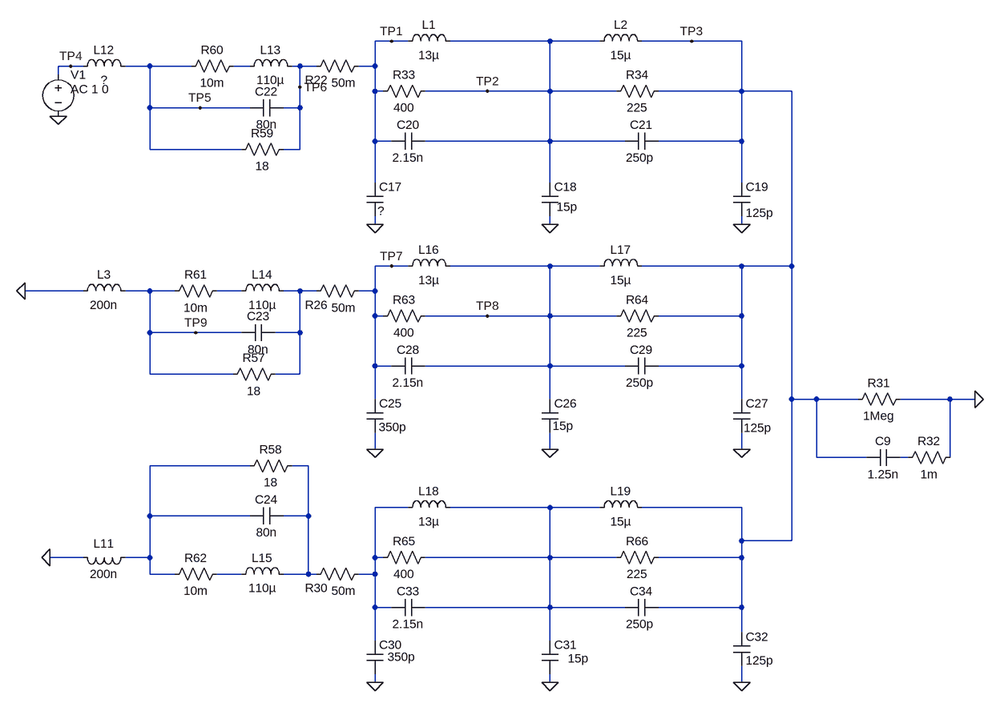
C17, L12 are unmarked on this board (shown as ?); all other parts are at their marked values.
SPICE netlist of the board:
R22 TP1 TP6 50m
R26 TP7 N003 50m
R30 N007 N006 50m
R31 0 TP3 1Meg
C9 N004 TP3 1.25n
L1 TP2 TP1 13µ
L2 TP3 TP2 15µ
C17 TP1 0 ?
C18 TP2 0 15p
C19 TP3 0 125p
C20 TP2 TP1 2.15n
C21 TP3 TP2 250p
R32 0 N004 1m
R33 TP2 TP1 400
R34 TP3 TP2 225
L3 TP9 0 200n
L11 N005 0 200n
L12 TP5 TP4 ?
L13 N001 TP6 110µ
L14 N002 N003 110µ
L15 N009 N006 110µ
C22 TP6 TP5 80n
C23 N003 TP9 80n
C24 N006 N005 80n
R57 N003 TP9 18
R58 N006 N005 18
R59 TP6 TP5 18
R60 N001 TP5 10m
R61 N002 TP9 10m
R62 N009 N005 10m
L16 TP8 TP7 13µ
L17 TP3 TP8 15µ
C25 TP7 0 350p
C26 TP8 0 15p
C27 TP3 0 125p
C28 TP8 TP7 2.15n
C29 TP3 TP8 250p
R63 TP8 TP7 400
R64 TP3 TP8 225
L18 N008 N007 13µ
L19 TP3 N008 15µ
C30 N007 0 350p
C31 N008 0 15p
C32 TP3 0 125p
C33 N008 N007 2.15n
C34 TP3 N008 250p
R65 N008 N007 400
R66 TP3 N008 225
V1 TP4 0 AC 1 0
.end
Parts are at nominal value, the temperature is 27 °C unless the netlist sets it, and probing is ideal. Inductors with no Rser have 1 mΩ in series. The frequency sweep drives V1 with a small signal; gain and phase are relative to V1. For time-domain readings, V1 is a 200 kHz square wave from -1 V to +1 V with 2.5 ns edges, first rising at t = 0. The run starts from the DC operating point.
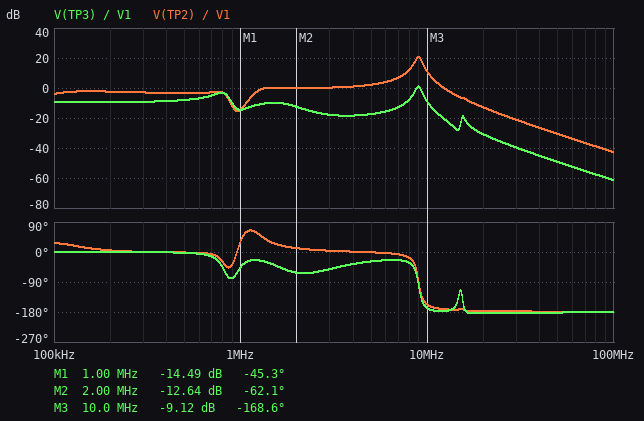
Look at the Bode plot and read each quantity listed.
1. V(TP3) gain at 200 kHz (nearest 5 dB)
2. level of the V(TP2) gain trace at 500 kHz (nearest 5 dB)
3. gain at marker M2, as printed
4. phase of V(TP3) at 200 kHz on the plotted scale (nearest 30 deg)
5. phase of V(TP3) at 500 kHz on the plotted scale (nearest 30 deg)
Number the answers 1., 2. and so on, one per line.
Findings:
1. -10 dB
2. -5 dB
3. -12.64 dB
4. 0 deg
5. 0 deg
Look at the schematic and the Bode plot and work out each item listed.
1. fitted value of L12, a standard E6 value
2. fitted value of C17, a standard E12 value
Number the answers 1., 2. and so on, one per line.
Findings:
1. 470 nH
2. 470 pF
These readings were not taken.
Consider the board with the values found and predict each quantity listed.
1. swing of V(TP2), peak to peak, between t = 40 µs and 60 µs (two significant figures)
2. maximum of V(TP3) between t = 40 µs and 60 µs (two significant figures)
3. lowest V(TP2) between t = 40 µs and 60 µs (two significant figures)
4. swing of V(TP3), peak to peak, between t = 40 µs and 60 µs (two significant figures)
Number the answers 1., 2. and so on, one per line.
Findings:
1. 5.2 V
2. 510 mV
3. -2.5 V
4. 1.0 V
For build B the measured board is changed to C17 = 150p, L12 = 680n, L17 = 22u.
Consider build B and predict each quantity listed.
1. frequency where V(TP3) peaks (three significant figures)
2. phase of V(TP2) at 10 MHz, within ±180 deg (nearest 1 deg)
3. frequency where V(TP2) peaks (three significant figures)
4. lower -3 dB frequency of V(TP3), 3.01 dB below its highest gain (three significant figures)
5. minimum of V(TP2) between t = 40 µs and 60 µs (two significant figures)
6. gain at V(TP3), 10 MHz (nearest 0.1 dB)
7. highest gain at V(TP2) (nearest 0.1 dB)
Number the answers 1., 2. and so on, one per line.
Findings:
1. 787 kHz
2. -68 deg
3. 10.2 MHz
4. 637 kHz
5. -2.4 V
6. -3.8 dB
7. 16.5 dB
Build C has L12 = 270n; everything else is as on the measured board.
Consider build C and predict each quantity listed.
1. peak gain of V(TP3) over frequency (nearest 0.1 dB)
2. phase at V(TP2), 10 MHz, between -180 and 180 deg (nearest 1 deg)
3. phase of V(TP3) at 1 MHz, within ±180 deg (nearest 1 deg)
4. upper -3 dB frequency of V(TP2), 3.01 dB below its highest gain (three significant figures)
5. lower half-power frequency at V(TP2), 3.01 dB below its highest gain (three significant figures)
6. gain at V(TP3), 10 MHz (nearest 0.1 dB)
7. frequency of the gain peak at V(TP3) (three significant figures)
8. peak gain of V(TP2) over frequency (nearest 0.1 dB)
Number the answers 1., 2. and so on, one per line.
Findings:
1. 2.6 dB
2. -9 deg
3. -45 deg
4. 12.2 MHz
5. 11.4 MHz
6. -10.1 dB
7. 11.8 MHz
8. 22.9 dB
